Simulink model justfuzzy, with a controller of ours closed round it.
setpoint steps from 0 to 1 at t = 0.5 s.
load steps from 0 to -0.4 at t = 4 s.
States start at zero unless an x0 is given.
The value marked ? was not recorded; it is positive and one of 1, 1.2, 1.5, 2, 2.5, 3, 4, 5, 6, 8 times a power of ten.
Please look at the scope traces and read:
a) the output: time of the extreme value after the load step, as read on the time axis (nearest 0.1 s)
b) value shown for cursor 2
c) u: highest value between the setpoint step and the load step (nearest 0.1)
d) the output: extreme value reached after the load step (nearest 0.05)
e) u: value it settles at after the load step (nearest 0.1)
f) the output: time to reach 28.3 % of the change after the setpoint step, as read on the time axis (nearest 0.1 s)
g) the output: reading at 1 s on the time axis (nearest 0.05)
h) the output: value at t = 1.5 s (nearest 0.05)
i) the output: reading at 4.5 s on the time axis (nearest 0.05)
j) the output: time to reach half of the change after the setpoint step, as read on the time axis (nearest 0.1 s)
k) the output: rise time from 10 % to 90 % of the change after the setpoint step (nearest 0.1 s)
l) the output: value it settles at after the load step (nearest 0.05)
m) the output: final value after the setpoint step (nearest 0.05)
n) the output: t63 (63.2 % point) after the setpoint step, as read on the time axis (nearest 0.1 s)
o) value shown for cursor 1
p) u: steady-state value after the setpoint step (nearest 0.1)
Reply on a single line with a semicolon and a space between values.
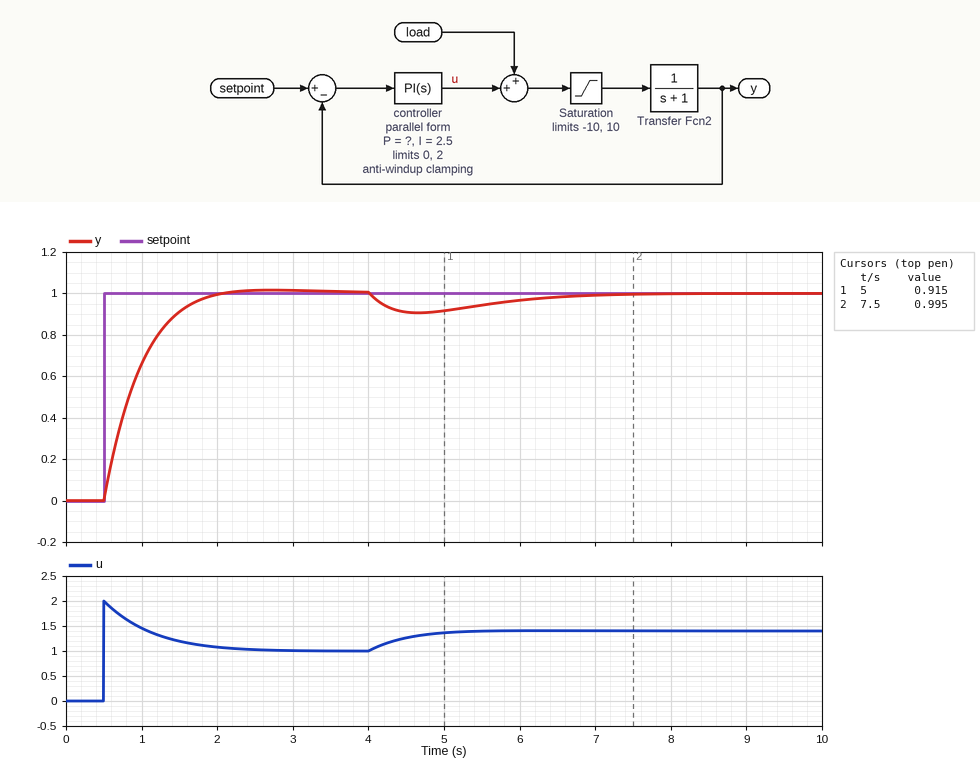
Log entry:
4.7 s; 0.995; 2.0; 0.90; 1.4; 0.7 s; 0.65; 0.90; 0.90; 0.8 s; 0.9 s; 1.00; 1.00; 1.0 s; 0.915; 1.0
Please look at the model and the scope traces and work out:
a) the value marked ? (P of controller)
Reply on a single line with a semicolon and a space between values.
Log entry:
2
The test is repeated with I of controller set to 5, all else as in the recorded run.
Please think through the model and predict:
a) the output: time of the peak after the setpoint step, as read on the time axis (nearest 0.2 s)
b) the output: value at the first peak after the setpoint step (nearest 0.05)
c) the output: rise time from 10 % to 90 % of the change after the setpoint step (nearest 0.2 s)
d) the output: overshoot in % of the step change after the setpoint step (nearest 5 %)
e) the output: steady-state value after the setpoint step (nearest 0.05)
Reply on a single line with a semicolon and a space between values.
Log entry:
1.8 s; 1.10; 0.6 s; 10 %; 1.00
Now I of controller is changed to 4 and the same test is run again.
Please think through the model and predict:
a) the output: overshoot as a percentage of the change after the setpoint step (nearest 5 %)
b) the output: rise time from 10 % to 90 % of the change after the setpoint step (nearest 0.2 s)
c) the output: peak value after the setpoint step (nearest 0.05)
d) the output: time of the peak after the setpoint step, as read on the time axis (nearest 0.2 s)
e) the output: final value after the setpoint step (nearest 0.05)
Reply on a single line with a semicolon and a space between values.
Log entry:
10 %; 0.6 s; 1.10; 2.0 s; 1.00
